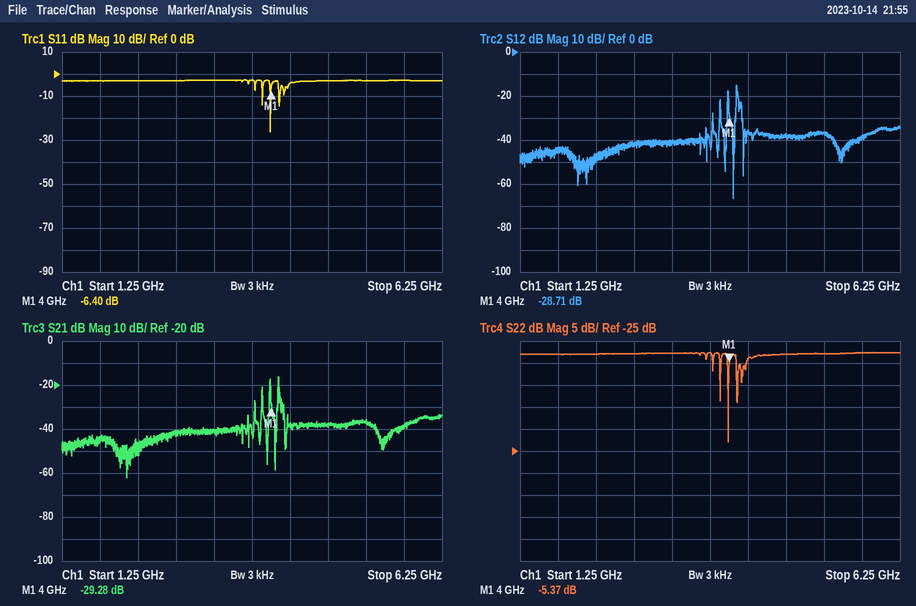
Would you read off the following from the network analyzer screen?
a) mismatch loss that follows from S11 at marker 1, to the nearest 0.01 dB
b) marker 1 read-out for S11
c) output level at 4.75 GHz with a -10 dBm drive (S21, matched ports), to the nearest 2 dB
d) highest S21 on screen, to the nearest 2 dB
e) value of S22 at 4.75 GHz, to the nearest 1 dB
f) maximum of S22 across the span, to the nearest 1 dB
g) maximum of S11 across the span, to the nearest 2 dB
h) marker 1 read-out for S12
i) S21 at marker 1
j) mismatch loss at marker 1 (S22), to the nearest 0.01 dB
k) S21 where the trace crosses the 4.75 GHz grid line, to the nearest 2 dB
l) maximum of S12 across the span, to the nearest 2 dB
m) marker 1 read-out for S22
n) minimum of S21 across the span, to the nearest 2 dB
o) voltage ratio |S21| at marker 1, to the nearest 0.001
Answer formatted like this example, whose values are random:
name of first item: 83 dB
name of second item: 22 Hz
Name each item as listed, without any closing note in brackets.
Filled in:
mismatch loss that follows from S11 at marker 1, to the nearest 0.01 dB: 1.13 dB
marker 1 read-out for S11: -6.40 dB
output level at 4.75 GHz with a -10 dBm drive (S21, matched ports), to the nearest 2 dB: -48 dBm
highest S21 on screen, to the nearest 2 dB: -16 dB
value of S22 at 4.75 GHz, to the nearest 1 dB: -3 dB
maximum of S22 across the span, to the nearest 1 dB: -3 dB
maximum of S11 across the span, to the nearest 2 dB: -2 dB
marker 1 read-out for S12: -28.71 dB
S21 at marker 1: -29.28 dB
mismatch loss at marker 1 (S22), to the nearest 0.01 dB: 1.49 dB
S21 where the trace crosses the 4.75 GHz grid line, to the nearest 2 dB: -38 dB
maximum of S12 across the span, to the nearest 2 dB: -16 dB
marker 1 read-out for S22: -5.37 dB
minimum of S21 across the span, to the nearest 2 dB: -62 dB
voltage ratio |S21| at marker 1, to the nearest 0.001: 0.034
